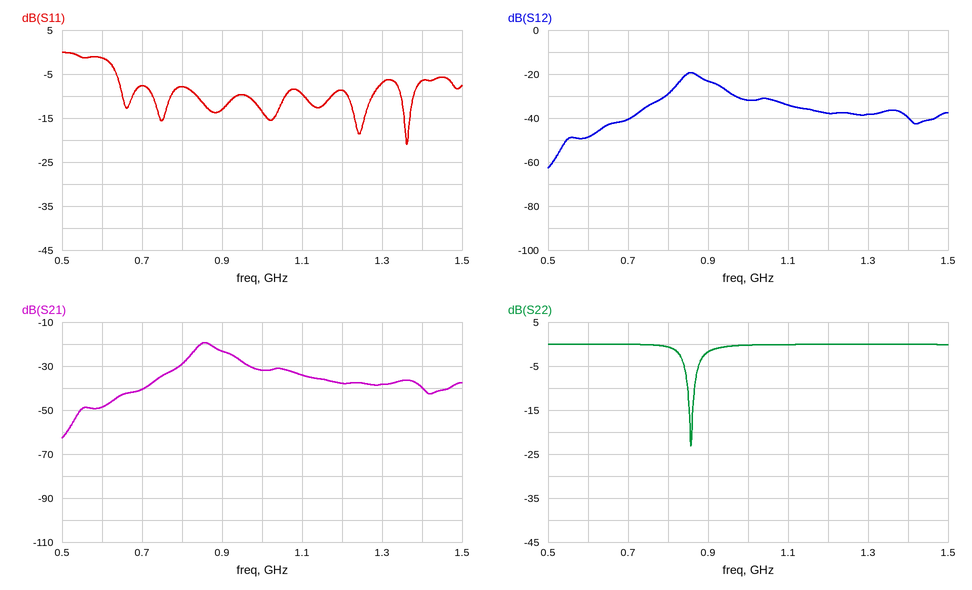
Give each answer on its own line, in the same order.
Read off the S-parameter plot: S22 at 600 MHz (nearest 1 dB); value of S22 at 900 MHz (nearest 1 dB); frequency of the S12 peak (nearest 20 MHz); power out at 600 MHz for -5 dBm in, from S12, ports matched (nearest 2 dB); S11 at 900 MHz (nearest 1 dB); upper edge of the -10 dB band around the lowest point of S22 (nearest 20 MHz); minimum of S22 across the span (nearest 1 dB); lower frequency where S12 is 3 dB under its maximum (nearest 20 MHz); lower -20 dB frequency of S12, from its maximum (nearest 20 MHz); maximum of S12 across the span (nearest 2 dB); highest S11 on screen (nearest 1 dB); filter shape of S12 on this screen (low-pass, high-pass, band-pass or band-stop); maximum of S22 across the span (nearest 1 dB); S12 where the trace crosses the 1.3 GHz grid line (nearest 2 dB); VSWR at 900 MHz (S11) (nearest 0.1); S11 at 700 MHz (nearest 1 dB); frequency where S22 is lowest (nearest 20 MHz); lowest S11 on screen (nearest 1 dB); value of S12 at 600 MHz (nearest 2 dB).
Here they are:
0 dB
-2 dB
860 MHz
-54 dBm
-13 dB
860 MHz
-23 dB
840 MHz
720 MHz
-20 dB
0 dB
band-pass
0 dB
-38 dB
1.6
-8 dB
860 MHz
-21 dB
-48 dB
